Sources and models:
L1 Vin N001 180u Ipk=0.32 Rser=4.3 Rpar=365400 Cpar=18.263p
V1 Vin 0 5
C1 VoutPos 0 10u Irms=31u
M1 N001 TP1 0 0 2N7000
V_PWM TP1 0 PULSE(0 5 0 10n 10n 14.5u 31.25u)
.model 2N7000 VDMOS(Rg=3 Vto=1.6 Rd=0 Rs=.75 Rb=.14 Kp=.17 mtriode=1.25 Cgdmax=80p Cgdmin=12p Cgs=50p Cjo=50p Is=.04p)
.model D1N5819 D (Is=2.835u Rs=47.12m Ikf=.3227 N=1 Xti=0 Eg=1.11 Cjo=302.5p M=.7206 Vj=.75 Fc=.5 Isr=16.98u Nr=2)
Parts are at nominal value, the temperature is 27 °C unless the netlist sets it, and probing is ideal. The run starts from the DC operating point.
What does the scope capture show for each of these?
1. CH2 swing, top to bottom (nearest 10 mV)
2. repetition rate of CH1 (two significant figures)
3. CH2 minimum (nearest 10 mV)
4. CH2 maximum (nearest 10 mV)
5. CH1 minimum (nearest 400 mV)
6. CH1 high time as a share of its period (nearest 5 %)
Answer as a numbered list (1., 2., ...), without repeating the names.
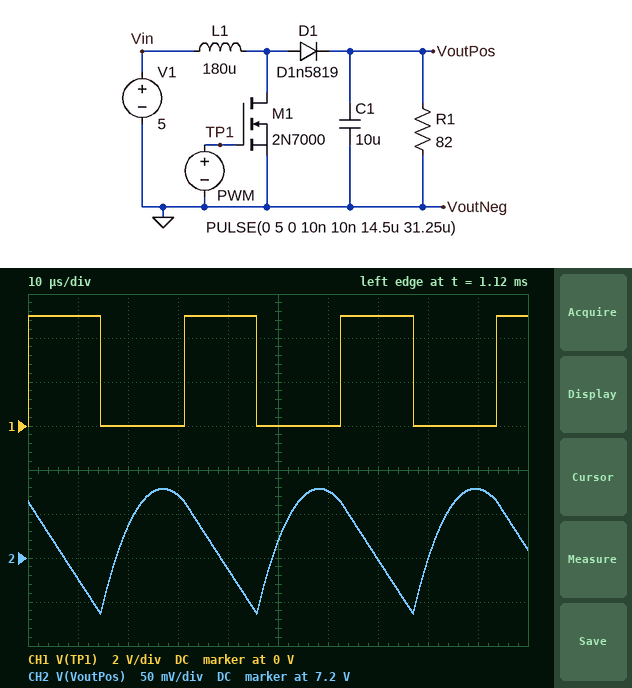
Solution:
1. 140 mV
2. 32 kHz
3. 7.14 V
4. 7.28 V
5. 0 V
6. 45 %
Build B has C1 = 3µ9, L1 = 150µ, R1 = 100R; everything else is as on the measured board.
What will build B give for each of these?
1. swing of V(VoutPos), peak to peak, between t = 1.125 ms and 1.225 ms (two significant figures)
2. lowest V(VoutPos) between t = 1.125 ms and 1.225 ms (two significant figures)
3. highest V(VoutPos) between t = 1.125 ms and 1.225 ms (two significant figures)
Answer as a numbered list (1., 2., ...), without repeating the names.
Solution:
1. 370 mV
2. 7.4 V
3. 7.8 V
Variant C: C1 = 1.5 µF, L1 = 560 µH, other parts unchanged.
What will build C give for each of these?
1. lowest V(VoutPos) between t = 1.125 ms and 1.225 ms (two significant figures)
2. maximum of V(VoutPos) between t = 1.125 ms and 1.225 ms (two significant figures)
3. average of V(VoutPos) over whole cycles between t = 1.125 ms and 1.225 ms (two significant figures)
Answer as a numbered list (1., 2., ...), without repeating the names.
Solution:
1. 6.8 V
2. 7.7 V
3. 7.3 V
